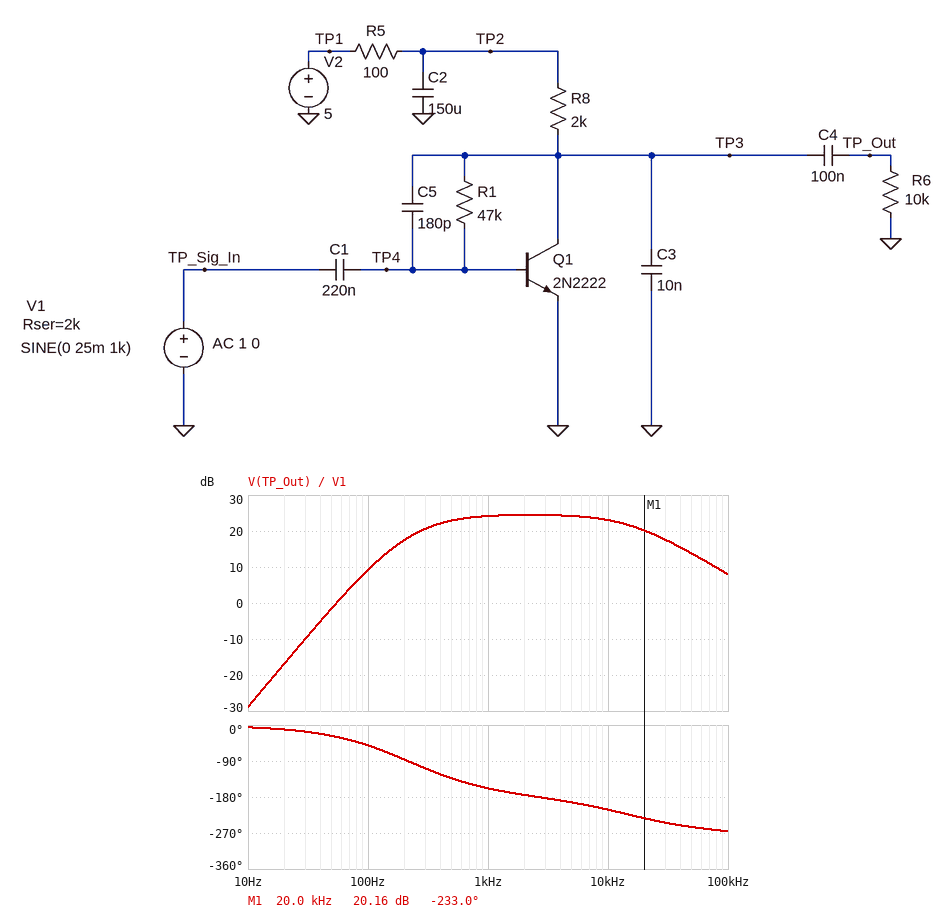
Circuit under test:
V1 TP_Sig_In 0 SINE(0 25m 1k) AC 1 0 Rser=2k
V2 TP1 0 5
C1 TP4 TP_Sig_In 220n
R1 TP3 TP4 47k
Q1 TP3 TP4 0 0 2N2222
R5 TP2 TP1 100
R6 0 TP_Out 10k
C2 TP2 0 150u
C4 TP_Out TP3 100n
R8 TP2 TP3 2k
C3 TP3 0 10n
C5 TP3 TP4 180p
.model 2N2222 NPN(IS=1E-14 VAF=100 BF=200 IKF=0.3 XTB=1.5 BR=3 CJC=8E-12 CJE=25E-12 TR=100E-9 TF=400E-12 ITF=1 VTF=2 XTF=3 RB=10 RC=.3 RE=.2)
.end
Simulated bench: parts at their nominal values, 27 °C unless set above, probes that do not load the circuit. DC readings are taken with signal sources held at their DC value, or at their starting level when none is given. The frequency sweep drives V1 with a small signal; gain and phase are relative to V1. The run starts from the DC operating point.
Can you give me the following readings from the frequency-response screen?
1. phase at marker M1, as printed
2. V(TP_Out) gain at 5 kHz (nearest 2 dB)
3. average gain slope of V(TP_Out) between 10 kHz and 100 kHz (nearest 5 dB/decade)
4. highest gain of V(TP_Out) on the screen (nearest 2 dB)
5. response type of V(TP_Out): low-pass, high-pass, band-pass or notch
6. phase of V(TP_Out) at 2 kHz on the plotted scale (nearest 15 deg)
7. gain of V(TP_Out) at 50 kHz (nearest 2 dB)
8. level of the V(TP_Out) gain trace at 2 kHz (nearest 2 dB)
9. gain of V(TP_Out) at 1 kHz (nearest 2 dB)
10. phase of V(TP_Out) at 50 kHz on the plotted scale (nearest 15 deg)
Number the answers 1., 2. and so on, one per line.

1. -233.0 deg
2. 24 dB
3. -15 dB/decade
4. 24 dB
5. band-pass
6. -180 deg
7. 14 dB
8. 24 dB
9. 24 dB
10. -255 deg
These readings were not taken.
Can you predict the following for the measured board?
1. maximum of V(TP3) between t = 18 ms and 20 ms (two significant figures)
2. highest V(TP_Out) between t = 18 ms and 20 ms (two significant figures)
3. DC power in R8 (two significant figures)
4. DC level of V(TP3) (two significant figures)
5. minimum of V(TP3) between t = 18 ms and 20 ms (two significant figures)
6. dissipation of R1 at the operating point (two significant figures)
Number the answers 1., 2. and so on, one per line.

1. 1.5 V
2. 400 mV
3. 6.9 mW
4. 1.1 V
5. 700 mV
6. 4.0 µW
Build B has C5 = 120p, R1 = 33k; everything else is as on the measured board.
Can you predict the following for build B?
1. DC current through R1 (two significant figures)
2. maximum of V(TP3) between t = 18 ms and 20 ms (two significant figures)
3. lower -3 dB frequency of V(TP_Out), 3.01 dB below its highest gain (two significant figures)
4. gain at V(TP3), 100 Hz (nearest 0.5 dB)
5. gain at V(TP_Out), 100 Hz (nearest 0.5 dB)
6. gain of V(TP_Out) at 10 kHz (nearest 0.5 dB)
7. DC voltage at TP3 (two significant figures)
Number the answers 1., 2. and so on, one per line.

1. 9.5 µA
2. 1.3 V
3. 370 Hz
4. 12.0 dB
5. 6.5 dB
6. 21.5 dB
7. 990 mV
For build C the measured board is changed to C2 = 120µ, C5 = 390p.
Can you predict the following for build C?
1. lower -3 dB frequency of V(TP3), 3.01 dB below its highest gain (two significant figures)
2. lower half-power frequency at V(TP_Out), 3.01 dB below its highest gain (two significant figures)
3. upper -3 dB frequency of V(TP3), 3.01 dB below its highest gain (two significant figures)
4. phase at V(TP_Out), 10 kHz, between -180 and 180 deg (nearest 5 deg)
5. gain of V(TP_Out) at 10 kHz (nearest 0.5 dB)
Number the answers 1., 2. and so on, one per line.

1. 280 Hz
2. 340 Hz
3. 9.4 kHz
4. 135 deg
5. 21.0 dB
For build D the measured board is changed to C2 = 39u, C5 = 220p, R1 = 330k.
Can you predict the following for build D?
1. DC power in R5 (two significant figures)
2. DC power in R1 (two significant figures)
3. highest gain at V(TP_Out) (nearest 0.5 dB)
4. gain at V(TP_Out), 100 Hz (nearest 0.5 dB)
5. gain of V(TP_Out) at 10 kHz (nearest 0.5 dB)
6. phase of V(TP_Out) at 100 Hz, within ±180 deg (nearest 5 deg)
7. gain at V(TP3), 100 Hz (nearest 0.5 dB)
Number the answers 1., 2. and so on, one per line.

1. 140 µW
2. 11 µW
3. 31.0 dB
4. 21.0 dB
5. 25.0 dB
6. -65 deg
7. 26.5 dB
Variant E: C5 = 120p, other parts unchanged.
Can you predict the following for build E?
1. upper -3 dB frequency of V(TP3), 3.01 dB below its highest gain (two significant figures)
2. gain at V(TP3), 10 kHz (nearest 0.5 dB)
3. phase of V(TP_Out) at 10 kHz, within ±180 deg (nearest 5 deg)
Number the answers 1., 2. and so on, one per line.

1. 19 kHz
2. 23.5 dB
3. 155 deg
